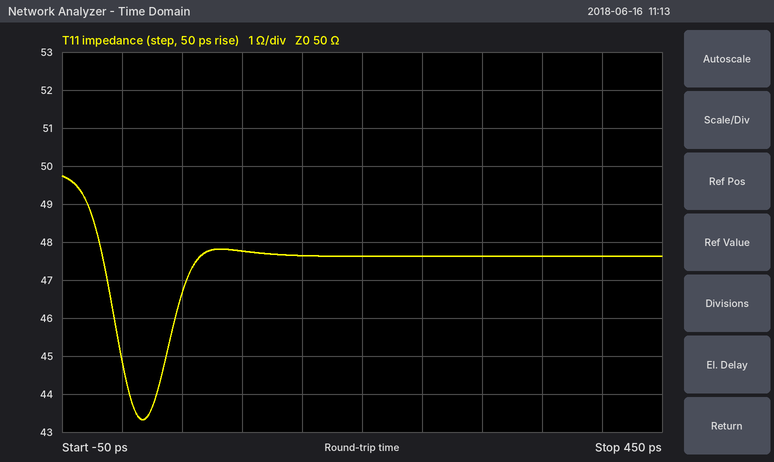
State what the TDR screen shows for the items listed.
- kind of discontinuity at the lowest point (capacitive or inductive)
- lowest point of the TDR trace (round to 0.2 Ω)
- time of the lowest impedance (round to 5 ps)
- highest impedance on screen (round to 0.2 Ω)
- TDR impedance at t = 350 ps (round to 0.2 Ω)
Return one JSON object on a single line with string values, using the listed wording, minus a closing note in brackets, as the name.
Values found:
{"kind of discontinuity at the lowest point": "capacitive", "lowest point of the TDR trace": "43.4 Ω", "time of the lowest impedance": "15 ps", "highest impedance on screen": "49.8 Ω", "TDR impedance at t = 350 ps": "47.6 Ω"}
